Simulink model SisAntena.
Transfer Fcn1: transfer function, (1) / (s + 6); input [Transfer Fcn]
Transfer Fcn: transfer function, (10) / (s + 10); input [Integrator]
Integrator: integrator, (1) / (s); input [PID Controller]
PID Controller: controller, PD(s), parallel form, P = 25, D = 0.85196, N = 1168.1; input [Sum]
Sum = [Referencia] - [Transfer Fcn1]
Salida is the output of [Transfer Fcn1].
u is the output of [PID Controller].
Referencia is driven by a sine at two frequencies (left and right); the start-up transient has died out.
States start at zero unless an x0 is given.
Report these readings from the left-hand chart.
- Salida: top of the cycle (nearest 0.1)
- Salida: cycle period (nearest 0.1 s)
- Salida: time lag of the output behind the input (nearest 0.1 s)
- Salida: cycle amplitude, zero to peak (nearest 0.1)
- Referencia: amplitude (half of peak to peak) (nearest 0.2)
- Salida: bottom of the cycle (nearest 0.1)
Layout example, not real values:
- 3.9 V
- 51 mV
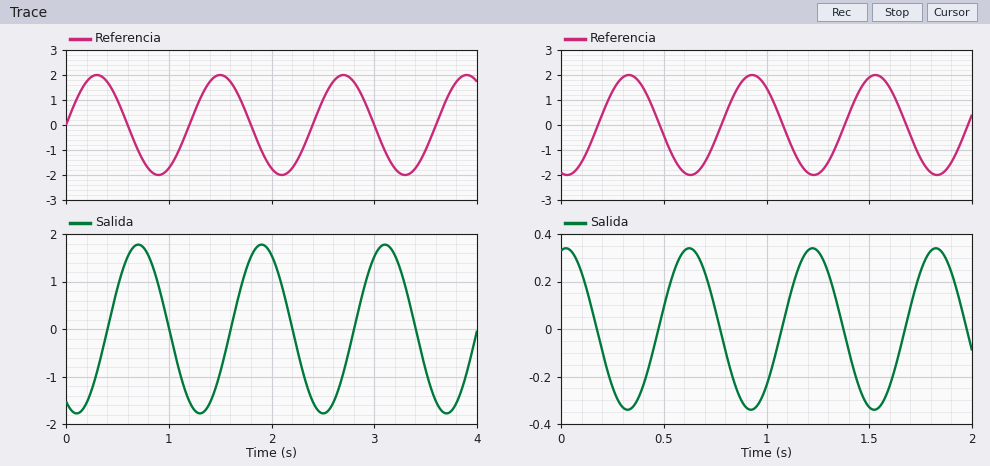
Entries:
- 1.8
- 1.2 s
- 0.4 s
- 1.8
- 2.0
- -1.8
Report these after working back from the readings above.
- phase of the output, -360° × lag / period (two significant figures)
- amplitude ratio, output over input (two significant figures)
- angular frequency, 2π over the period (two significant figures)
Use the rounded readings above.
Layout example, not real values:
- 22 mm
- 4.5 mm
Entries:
- -120°
- 0.90
- 5.2 rad/s
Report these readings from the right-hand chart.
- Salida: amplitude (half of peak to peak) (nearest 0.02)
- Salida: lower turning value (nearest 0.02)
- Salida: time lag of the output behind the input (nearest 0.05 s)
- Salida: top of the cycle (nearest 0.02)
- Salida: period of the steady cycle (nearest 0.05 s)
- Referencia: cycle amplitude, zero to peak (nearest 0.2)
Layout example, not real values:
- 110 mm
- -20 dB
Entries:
- 0.34
- -0.34
- 0.30 s
- 0.34
- 0.60 s
- 2.0
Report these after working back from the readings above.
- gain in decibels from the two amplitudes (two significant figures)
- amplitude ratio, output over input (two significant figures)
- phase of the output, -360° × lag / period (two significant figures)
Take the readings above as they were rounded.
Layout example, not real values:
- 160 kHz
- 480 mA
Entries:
- -15 dB
- 0.17
- -180°
